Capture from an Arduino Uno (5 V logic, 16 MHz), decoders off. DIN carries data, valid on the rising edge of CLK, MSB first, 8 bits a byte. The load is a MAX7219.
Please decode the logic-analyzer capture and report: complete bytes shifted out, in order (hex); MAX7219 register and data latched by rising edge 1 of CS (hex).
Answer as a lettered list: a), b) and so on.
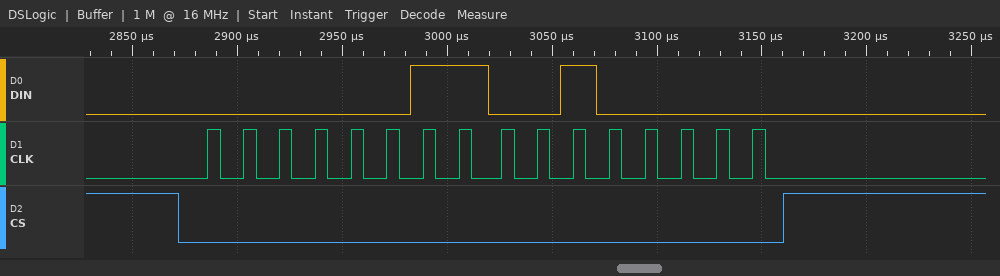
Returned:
a) 0x03 0x20
b) register 0x3, data 0x20
